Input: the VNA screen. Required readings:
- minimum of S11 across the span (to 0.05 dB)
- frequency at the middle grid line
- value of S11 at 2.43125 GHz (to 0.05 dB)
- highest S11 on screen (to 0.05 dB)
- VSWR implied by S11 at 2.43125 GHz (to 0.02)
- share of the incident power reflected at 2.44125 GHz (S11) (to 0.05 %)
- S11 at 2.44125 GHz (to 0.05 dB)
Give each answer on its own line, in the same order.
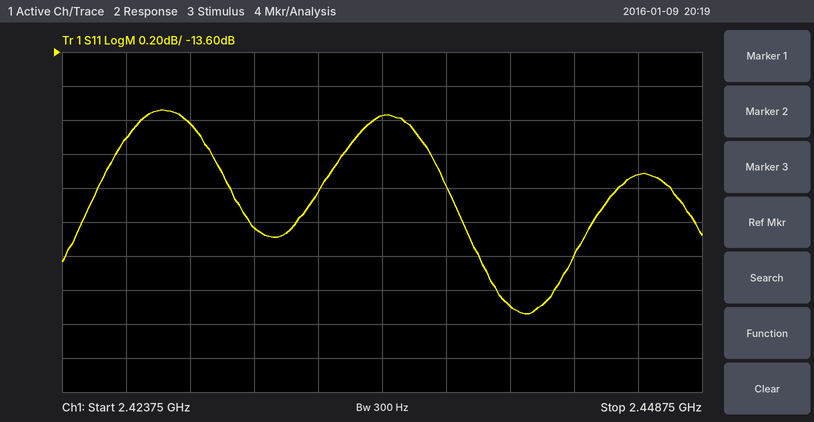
-15.15 dB
2.43625 GHz
-14.65 dB
-13.95 dB
1.46
3.10 %
-15.10 dB
